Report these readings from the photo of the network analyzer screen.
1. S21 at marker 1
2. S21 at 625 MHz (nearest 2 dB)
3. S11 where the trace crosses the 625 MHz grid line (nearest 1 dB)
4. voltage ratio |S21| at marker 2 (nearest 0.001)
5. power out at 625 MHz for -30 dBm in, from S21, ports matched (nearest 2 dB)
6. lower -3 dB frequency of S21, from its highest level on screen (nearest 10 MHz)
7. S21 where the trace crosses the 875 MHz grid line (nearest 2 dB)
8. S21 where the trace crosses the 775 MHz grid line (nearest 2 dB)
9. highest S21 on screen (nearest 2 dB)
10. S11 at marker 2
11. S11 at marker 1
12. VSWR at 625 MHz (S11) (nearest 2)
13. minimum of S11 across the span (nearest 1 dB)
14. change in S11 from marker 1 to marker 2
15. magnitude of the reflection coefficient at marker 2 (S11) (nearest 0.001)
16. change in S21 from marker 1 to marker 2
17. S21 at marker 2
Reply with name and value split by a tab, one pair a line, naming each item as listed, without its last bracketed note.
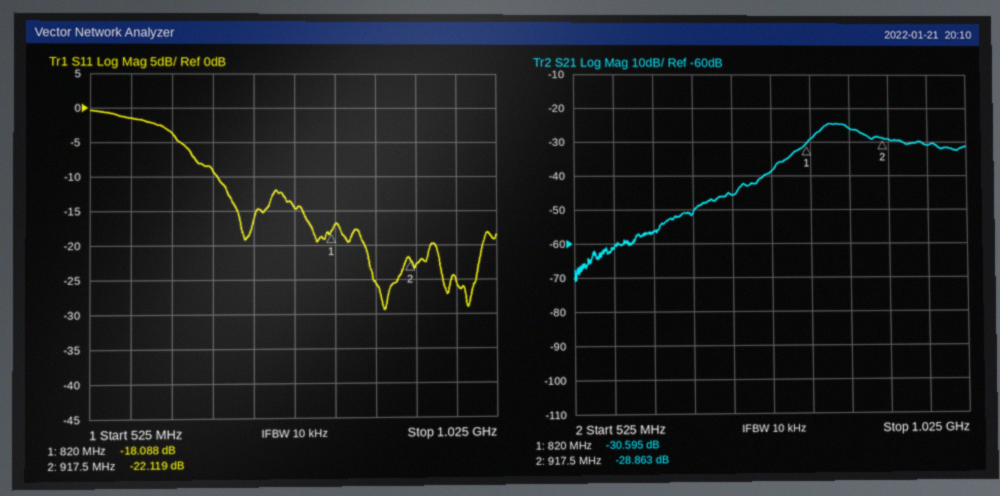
S21 at marker 1	-30.595 dB
S21 at 625 MHz	-56 dB
S11 where the trace crosses the 625 MHz grid line	-4 dB
voltage ratio |S21| at marker 2	0.036
power out at 625 MHz for -30 dBm in, from S21, ports matched	-86 dBm
lower -3 dB frequency of S21, from its highest level on screen	830 MHz
S21 where the trace crosses the 875 MHz grid line	-26 dB
S21 where the trace crosses the 775 MHz grid line	-38 dB
highest S21 on screen	-24 dB
S11 at marker 2	-22.119 dB
S11 at marker 1	-18.088 dB
VSWR at 625 MHz (S11)	4
minimum of S11 across the span	-29 dB
change in S11 from marker 1 to marker 2	-4.031 dB
magnitude of the reflection coefficient at marker 2 (S11)	0.078
change in S21 from marker 1 to marker 2	1.732 dB
S21 at marker 2	-28.863 dB
